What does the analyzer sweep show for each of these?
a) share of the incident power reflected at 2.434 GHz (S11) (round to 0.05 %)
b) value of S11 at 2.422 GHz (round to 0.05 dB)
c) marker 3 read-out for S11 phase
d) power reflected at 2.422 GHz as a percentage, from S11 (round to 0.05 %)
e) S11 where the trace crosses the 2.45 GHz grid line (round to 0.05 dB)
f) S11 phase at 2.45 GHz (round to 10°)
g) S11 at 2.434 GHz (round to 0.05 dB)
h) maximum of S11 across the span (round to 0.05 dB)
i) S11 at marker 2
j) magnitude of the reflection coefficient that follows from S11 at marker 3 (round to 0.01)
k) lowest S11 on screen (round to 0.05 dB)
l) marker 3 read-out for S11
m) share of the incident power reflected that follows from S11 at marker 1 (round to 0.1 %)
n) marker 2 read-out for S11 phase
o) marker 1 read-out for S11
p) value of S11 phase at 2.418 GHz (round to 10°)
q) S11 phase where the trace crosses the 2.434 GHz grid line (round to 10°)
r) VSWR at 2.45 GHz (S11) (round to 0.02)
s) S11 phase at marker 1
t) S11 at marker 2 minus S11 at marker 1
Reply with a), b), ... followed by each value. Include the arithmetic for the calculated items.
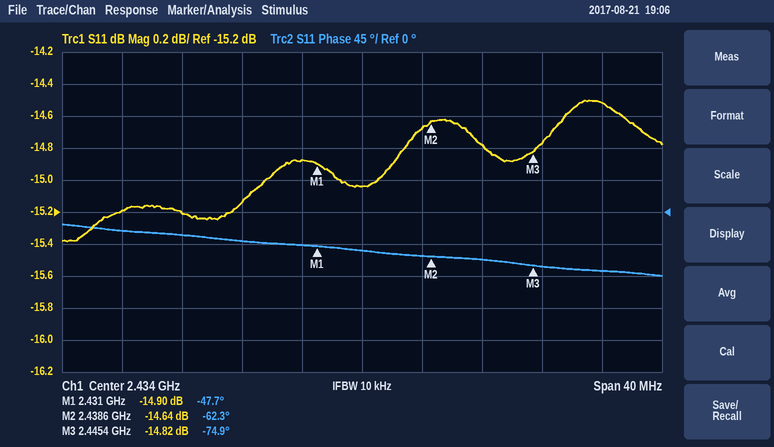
a) 10^(-15.05/10) ≈ 3.13 %, so 3.15 % to the nearest 0.05 %
b) -15.20 dB
c) -74.9°
d) 10^(-15.2/10) ≈ 3.02 %, so 3.00 % to the nearest 0.05 %
e) -14.50 dB
f) -80°
g) -15.05 dB
h) -14.50 dB
i) -14.64 dB
j) 10^(-14.82/20) ≈ 0.18
k) -15.40 dB
l) -14.82 dB
m) 10^(-14.9/10) ≈ 3.2 %
n) -62.3°
o) -14.90 dB
p) -30°
q) -50°
r) |Γ| = 10^(-14.5/20) = 0.1884; VSWR = (1 + 0.1884)/(1 − 0.1884) ≈ 1.46
s) -47.7°
t) -14.64 − (-14.9) = 0.26 dB
